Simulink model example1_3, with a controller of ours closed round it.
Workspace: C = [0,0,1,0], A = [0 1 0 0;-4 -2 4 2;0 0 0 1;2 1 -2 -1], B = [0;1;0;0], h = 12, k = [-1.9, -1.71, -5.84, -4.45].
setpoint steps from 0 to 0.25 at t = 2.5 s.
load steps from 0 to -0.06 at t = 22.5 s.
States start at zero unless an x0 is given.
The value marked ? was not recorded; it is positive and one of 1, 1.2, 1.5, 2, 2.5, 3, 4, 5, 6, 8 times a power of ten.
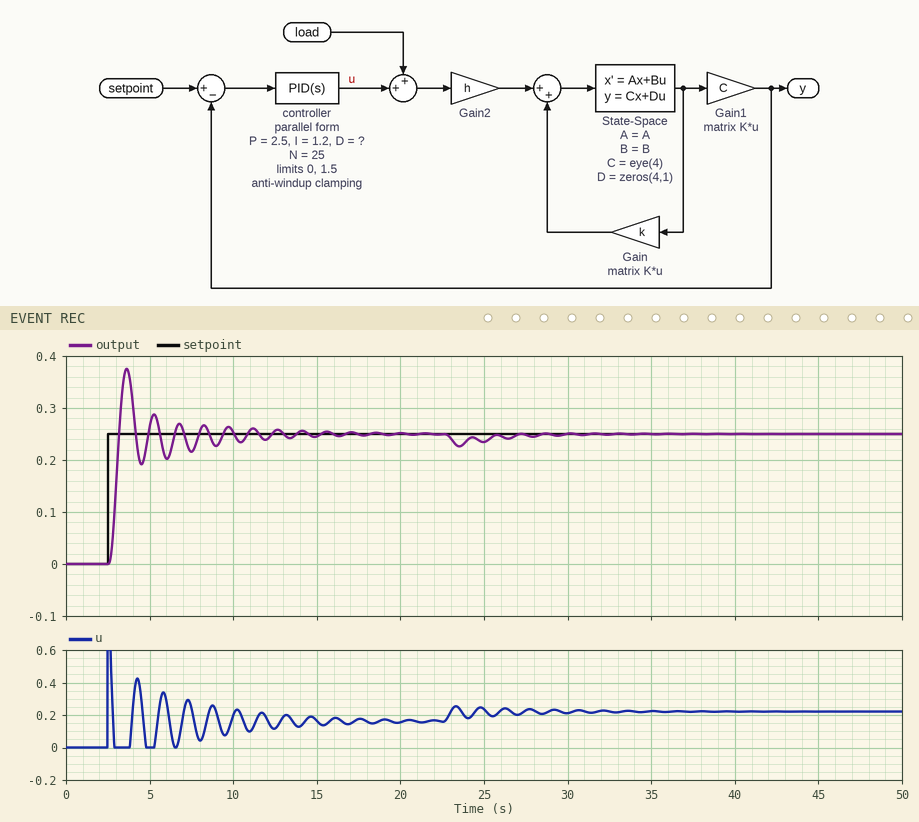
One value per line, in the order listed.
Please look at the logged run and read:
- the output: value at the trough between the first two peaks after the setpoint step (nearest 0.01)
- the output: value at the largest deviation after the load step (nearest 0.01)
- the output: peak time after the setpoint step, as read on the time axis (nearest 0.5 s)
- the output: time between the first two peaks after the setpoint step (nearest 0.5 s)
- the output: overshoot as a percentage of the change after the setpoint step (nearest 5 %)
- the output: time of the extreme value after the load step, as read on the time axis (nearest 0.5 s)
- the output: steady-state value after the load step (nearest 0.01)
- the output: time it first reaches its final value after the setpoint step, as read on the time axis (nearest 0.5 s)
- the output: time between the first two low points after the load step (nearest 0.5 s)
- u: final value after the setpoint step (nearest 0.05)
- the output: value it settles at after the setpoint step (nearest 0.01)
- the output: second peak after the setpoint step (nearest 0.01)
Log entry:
0.19
0.23
3.5 s
1.5 s
50 %
23.5 s
0.25
3.0 s
1.5 s
0.15
0.25
0.29
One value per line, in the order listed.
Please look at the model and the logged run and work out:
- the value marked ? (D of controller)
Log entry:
1
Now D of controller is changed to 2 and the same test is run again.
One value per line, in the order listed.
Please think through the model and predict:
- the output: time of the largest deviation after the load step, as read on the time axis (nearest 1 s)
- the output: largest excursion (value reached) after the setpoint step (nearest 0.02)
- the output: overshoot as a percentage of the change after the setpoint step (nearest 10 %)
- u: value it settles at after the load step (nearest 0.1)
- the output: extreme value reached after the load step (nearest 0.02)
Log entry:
23 s
0.34
40 %
0.2
0.24
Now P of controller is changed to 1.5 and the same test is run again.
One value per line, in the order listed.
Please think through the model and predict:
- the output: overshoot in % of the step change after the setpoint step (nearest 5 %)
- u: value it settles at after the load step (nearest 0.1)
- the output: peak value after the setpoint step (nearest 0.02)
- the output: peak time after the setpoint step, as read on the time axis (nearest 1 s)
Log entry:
20 %
0.2
0.30
4 s
